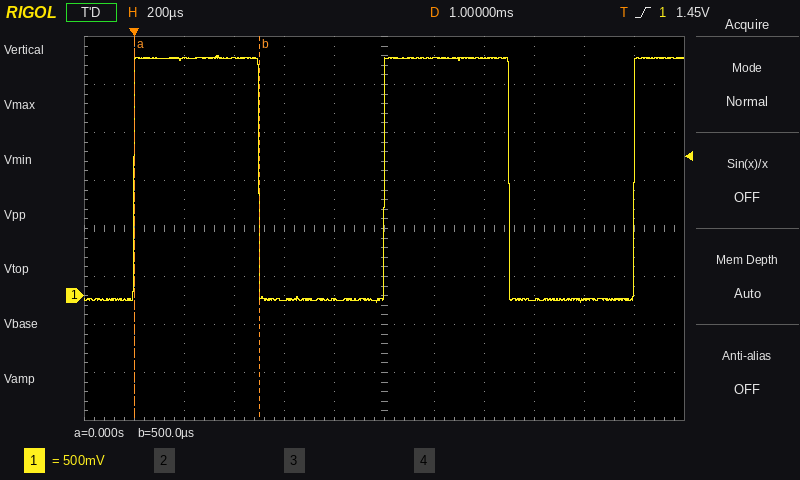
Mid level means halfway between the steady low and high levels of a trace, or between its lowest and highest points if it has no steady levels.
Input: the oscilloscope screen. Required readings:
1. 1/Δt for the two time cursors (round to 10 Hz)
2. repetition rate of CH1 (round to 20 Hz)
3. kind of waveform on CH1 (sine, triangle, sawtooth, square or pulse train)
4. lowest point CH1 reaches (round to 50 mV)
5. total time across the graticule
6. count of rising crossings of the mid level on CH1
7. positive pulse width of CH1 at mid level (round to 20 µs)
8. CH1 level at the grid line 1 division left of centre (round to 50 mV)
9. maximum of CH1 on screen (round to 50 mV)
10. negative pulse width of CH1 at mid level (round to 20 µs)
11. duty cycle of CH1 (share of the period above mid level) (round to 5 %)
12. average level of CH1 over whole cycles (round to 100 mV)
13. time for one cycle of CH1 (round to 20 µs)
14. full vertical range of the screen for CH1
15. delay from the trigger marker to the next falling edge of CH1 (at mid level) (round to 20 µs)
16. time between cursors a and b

2.00 kHz
1.00 kHz
square
-50 mV
2.4 ms
3
500 µs
-50 mV
2.50 V
500 µs
50 %
1.2 V
1.00 ms
4 V
500 µs
500 µs
